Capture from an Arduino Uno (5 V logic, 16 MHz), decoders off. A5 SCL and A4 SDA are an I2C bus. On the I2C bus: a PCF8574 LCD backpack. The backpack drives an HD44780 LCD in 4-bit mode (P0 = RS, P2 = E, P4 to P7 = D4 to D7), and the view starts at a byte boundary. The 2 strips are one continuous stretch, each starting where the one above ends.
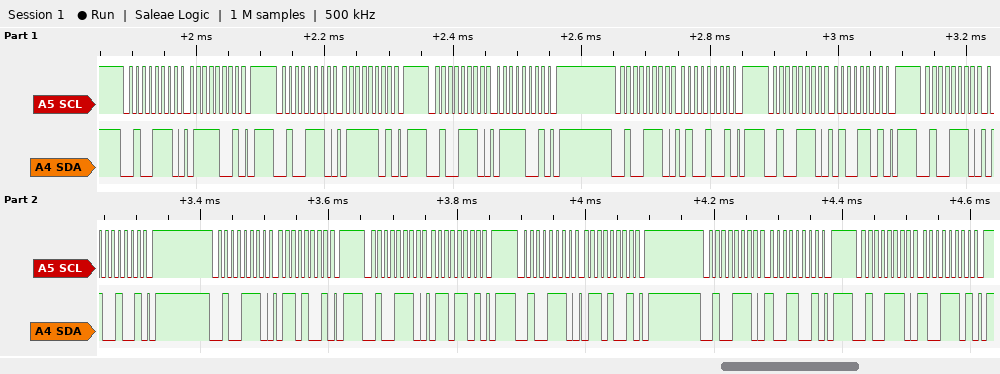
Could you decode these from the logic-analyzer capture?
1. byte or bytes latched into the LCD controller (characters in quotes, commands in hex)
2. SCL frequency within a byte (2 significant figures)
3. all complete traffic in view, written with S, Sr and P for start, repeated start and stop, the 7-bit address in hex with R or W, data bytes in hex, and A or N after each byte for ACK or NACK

't'
100 kHz
S 27W A 79 A P S 27W A 7D A P S 27W A 79 A P S 27W A 49 A P S 27W A 4D A P S 27W A 49 A P S 27W A 69 A P S 27W A 6D A P S 27W A 69 A P S 27W A 99 A P S 27W A 9D A P
